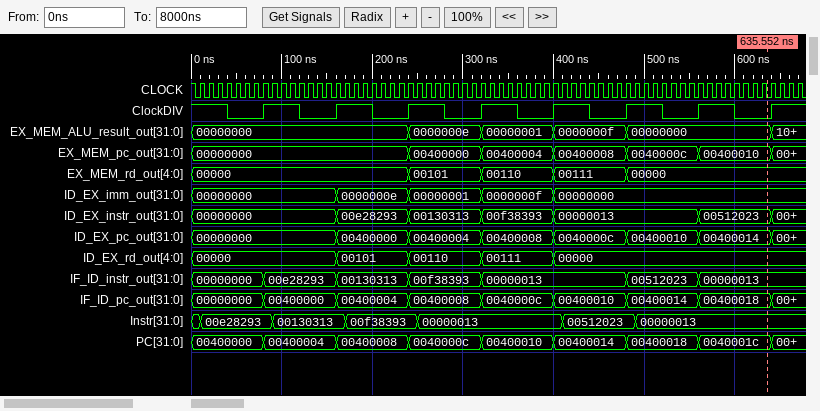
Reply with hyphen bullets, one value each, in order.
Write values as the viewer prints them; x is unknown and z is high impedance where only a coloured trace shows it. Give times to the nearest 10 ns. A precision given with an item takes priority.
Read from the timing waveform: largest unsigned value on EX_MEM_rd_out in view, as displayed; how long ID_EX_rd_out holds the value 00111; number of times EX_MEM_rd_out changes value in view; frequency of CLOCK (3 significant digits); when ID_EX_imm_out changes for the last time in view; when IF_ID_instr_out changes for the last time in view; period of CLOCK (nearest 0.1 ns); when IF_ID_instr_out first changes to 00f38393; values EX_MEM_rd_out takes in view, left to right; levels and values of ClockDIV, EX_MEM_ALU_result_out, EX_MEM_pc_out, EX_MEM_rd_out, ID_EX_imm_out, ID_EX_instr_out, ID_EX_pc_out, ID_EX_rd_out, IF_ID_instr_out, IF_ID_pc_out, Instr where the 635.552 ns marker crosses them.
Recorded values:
- 00111
- 80 ns
- 4
- 100 MHz
- 400 ns
- 560 ns
- 10 ns
- 240 ns
- 00000, 00101, 00110, 00111, 00000
- ClockDIV=0, EX_MEM_ALU_result_out=00000000, EX_MEM_pc_out=00400010, EX_MEM_rd_out=00000, ID_EX_imm_out=00000000, ID_EX_instr_out=00512023, ID_EX_pc_out=00400014, ID_EX_rd_out=00000, IF_ID_instr_out=00000013, IF_ID_pc_out=00400018, Instr=00000013
